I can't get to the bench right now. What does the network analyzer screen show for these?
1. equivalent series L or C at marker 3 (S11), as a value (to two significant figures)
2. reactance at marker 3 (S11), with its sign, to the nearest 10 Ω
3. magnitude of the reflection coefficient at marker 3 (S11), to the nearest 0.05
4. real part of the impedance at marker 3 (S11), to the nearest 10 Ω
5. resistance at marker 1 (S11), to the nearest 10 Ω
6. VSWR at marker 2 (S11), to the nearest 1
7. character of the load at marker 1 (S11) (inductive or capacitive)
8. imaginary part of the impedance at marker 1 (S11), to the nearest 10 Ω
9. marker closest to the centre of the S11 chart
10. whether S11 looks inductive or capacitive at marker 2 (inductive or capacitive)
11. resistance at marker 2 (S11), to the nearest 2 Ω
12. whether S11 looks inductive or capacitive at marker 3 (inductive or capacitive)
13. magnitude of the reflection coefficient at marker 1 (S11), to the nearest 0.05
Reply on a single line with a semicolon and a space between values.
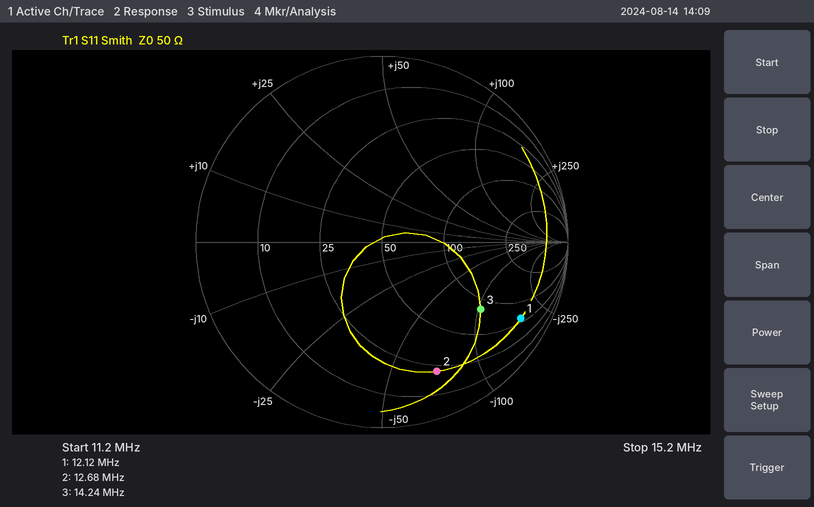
110 pF; -100 Ω; 0.65; 80 Ω; 60 Ω; 7; capacitive; -180 Ω; marker 3; capacitive; 22 Ω; capacitive; 0.85
